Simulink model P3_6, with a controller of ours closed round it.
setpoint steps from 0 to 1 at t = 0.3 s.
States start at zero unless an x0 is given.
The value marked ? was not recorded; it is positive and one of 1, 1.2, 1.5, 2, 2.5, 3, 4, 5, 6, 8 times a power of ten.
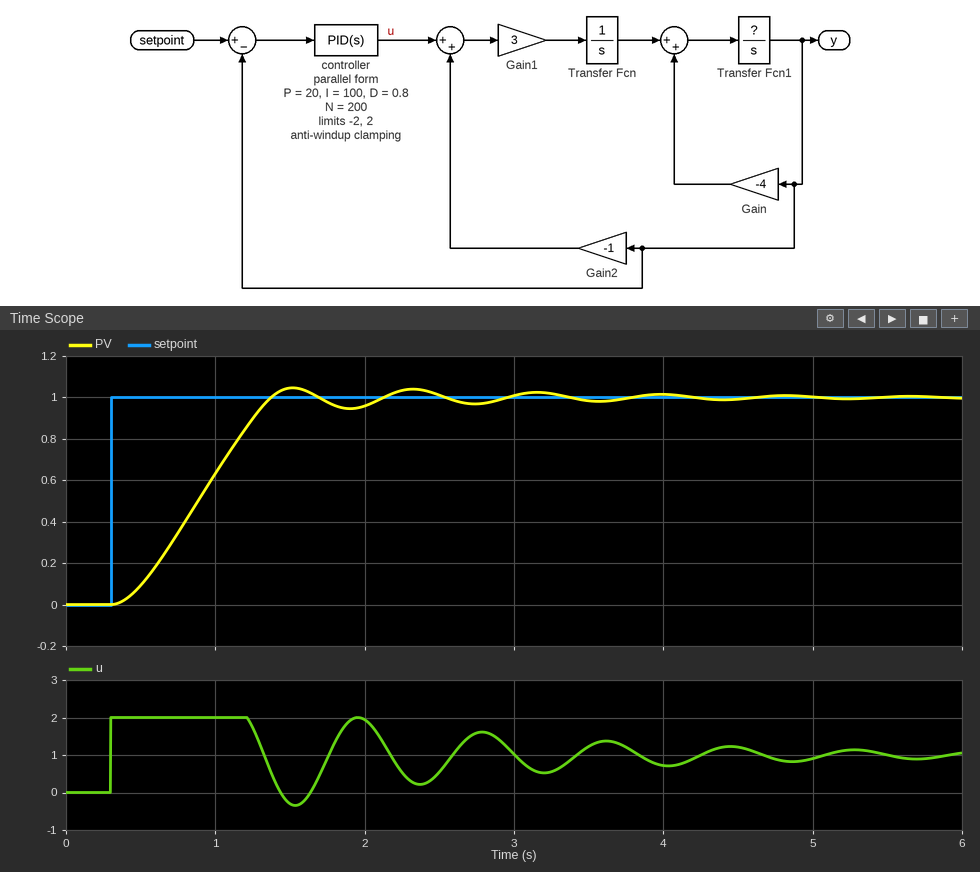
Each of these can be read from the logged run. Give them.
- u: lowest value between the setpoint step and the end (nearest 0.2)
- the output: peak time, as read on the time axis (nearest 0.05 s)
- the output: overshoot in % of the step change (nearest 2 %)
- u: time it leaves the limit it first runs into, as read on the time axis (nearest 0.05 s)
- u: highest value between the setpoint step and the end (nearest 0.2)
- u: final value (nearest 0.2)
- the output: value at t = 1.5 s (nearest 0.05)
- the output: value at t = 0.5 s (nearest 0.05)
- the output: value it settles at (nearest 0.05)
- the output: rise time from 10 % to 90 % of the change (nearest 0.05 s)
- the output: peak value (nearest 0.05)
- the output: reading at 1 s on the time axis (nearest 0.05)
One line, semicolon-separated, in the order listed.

-0.4; 1.50 s; 4 %; 1.20 s; 2.0; 1.0; 1.05; 0.10; 1.00; 0.75 s; 1.05; 0.65
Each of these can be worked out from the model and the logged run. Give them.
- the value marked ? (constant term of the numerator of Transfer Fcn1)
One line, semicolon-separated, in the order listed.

1
